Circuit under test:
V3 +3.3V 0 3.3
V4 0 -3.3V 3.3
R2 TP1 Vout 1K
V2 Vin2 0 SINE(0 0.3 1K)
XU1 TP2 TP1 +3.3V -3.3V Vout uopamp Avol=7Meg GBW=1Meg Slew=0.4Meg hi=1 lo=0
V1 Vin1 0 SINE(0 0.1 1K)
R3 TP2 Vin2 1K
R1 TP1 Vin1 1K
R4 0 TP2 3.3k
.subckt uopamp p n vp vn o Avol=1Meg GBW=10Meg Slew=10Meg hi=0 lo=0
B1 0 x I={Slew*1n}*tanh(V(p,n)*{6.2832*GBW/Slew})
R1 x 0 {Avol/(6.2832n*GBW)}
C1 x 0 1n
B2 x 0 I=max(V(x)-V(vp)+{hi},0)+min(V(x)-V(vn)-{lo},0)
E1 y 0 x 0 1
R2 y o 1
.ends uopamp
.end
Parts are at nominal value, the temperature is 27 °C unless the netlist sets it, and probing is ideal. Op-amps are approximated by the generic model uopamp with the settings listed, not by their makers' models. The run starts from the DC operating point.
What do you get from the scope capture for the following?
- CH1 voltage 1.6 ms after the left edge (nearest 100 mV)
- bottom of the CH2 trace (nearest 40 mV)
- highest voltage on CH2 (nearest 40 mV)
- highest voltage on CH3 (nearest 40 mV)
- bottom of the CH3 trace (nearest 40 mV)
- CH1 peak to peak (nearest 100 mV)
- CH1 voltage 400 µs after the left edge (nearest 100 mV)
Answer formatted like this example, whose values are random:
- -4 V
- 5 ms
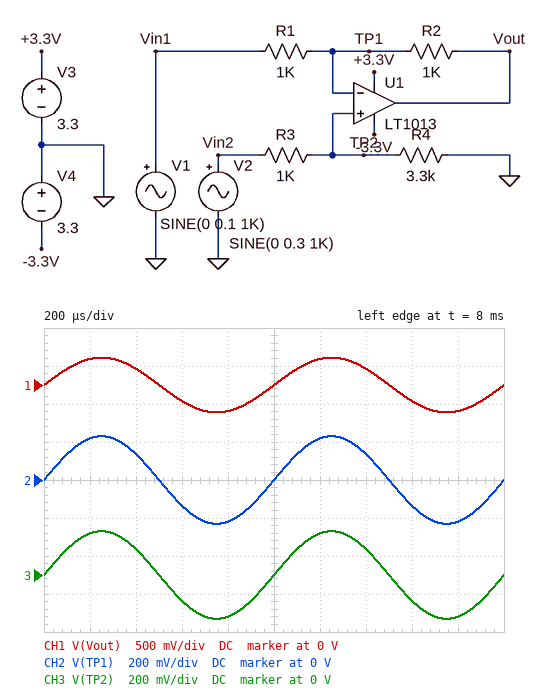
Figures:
- -200 mV
- -240 mV
- 240 mV
- 240 mV
- -240 mV
- 700 mV
- 200 mV
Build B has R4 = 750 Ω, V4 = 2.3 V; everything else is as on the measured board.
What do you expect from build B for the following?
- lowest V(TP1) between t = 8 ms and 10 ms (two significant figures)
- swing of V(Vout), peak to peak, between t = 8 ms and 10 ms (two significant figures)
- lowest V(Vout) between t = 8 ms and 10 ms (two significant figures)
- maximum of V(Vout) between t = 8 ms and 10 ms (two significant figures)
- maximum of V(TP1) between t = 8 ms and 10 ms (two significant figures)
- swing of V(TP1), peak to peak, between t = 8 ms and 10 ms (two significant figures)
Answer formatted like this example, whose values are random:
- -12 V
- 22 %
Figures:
- -130 mV
- 310 mV
- -160 mV
- 160 mV
- 130 mV
- 260 mV
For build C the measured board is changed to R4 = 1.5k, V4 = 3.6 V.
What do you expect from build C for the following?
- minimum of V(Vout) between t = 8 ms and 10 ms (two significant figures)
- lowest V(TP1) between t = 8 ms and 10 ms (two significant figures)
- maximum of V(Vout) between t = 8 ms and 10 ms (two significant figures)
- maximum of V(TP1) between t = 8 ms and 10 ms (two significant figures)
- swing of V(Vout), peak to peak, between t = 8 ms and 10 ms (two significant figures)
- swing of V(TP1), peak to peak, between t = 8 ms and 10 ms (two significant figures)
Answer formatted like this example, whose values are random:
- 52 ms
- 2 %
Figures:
- -260 mV
- -180 mV
- 260 mV
- 180 mV
- 520 mV
- 360 mV
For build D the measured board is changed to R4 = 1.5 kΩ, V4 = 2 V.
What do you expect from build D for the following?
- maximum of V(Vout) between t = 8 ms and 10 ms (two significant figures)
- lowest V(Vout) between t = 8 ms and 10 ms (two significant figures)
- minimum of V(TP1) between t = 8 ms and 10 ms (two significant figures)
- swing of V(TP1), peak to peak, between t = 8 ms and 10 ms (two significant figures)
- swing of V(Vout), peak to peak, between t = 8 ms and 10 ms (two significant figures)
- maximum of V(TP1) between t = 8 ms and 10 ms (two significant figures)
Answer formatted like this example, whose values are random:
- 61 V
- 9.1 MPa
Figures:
- 260 mV
- -260 mV
- -180 mV
- 360 mV
- 520 mV
- 180 mV
